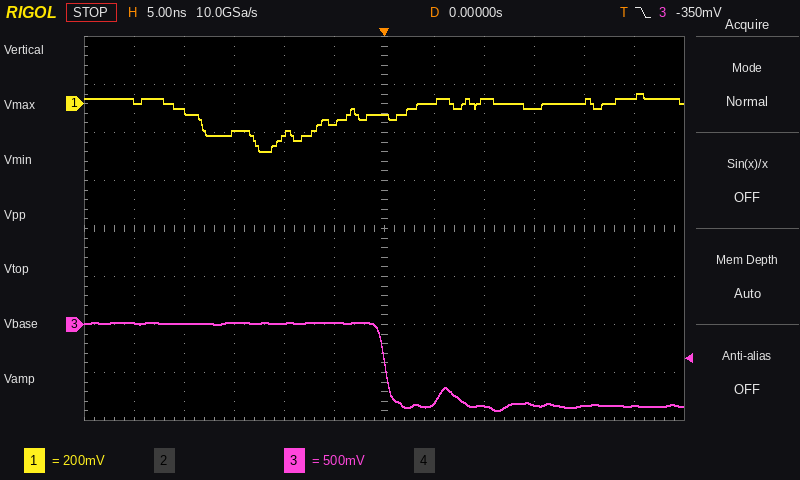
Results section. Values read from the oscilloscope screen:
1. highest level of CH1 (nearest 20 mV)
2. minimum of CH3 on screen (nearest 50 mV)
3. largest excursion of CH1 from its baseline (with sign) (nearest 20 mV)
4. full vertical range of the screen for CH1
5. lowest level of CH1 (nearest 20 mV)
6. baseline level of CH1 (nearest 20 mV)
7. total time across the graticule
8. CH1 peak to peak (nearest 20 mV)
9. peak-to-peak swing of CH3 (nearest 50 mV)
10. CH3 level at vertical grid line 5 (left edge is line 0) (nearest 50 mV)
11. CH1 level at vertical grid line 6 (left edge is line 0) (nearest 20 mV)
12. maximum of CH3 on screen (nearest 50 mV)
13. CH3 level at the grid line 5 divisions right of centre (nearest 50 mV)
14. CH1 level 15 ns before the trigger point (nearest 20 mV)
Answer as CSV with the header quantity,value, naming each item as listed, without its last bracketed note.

quantity,value
highest level of CH1,40 mV
minimum of CH3 on screen,-900 mV
largest excursion of CH1 from its baseline (with sign),-200 mV
full vertical range of the screen for CH1,1.6 V
lowest level of CH1,-200 mV
baseline level of CH1,0 mV
total time across the graticule,60 ns
CH1 peak to peak,240 mV
peak-to-peak swing of CH3,900 mV
CH3 level at vertical grid line 5 (left edge is line 0),0 mV
CH1 level at vertical grid line 6 (left edge is line 0),-40 mV
maximum of CH3 on screen,0 mV
CH3 level at the grid line 5 divisions right of centre,-850 mV
CH1 level 15 ns before the trigger point,-120 mV
